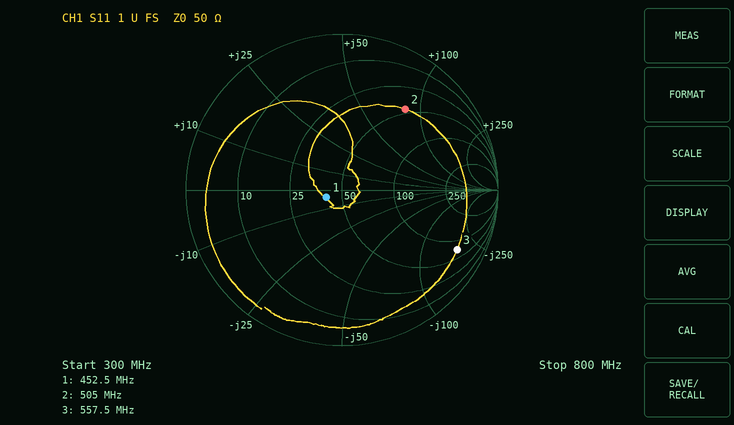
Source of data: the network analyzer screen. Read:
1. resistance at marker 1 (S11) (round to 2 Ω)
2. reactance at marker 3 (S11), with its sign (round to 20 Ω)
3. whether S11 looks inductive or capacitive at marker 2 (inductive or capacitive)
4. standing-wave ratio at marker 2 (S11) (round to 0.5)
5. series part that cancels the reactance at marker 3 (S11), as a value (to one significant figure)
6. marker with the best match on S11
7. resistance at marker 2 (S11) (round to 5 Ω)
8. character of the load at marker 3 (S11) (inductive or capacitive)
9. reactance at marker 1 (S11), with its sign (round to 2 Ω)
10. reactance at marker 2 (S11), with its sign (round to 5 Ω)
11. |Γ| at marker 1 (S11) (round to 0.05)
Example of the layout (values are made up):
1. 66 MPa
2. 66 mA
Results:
1. 40 Ω
2. -180 Ω
3. inductive
4. 5.0
5. 50 nH
6. marker 1
7. 45 Ω
8. capacitive
9. -4 Ω
10. +85 Ω
11. 0.10
